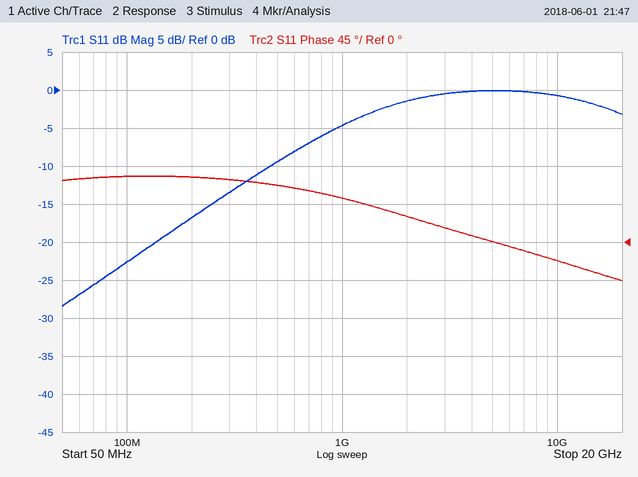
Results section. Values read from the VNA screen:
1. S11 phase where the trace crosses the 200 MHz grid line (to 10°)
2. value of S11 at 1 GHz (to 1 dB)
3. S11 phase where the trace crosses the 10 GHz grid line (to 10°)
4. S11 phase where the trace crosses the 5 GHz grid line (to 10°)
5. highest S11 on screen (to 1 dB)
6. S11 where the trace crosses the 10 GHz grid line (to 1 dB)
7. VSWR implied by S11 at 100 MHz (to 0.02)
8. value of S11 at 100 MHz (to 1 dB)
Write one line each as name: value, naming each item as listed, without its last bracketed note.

S11 phase where the trace crosses the 200 MHz grid line: 80°
value of S11 at 1 GHz: -5 dB
S11 phase where the trace crosses the 10 GHz grid line: -20°
S11 phase where the trace crosses the 5 GHz grid line: 0°
highest S11 on screen: 0 dB
S11 where the trace crosses the 10 GHz grid line: -1 dB
VSWR implied by S11 at 100 MHz: 1.16
value of S11 at 100 MHz: -23 dB
